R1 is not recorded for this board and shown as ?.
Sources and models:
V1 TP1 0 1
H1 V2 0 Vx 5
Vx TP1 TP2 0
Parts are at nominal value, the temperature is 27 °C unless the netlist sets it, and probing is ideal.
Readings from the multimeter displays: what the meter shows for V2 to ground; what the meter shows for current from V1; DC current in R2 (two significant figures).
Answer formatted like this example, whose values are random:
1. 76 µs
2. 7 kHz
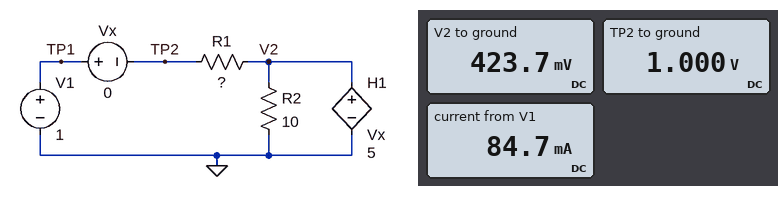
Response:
1. 423.7 mV
2. 84.7 mA
3. 42 mA
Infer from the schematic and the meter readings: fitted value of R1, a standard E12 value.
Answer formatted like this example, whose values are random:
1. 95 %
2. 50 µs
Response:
1. 6.8 Ω
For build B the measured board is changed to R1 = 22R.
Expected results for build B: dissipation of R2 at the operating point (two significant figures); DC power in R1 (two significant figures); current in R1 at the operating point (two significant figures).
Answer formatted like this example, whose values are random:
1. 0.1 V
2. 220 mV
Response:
1. 3.4 mW
2. 30 mW
3. 37 mA
